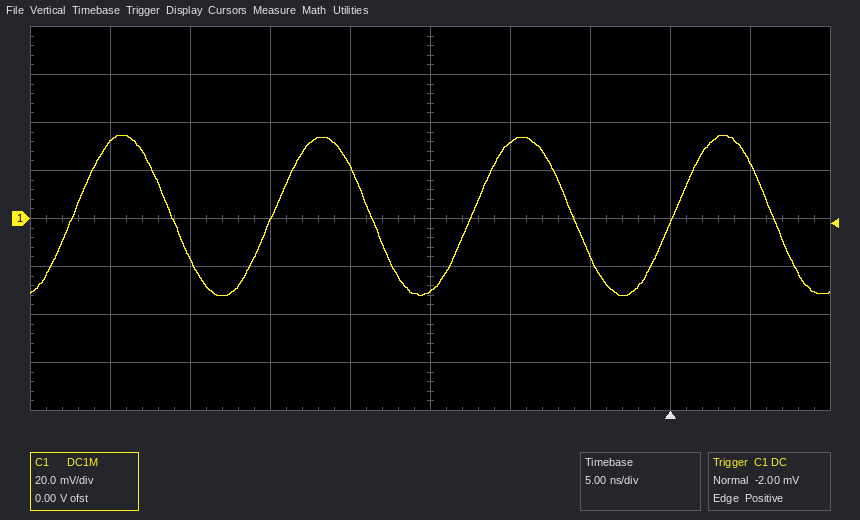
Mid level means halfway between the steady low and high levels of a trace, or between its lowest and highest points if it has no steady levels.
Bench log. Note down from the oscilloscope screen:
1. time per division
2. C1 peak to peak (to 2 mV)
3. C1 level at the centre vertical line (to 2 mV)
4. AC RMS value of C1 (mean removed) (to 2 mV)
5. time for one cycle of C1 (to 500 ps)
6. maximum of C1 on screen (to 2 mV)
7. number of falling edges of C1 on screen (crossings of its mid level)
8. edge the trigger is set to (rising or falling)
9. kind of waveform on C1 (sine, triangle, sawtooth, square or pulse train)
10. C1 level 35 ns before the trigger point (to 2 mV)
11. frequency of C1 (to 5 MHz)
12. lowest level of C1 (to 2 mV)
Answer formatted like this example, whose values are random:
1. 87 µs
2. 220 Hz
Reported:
1. 5 ns
2. 66 mV
3. -30 mV
4. 24 mV
5. 12.5 ns
6. 34 mV
7. 4
8. rising
9. sine
10. 32 mV
11. 80 MHz
12. -32 mV
